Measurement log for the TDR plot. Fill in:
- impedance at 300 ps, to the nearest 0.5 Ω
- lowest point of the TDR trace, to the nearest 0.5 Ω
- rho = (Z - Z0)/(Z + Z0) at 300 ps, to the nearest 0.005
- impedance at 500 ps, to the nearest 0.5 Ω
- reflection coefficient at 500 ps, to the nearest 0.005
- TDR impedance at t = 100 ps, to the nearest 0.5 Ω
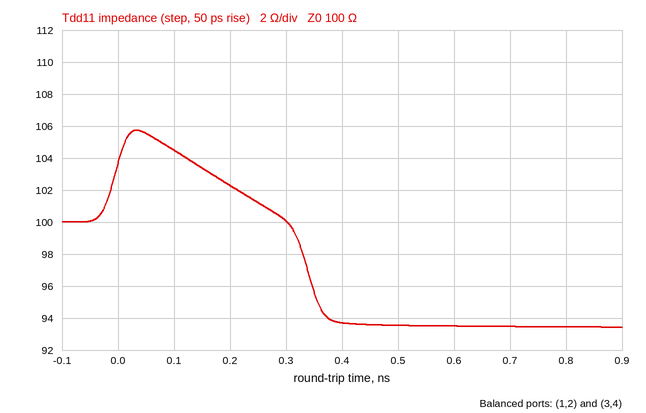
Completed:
100.0 Ω
93.5 Ω
0.000
93.5 Ω
-0.035
104.5 Ω
